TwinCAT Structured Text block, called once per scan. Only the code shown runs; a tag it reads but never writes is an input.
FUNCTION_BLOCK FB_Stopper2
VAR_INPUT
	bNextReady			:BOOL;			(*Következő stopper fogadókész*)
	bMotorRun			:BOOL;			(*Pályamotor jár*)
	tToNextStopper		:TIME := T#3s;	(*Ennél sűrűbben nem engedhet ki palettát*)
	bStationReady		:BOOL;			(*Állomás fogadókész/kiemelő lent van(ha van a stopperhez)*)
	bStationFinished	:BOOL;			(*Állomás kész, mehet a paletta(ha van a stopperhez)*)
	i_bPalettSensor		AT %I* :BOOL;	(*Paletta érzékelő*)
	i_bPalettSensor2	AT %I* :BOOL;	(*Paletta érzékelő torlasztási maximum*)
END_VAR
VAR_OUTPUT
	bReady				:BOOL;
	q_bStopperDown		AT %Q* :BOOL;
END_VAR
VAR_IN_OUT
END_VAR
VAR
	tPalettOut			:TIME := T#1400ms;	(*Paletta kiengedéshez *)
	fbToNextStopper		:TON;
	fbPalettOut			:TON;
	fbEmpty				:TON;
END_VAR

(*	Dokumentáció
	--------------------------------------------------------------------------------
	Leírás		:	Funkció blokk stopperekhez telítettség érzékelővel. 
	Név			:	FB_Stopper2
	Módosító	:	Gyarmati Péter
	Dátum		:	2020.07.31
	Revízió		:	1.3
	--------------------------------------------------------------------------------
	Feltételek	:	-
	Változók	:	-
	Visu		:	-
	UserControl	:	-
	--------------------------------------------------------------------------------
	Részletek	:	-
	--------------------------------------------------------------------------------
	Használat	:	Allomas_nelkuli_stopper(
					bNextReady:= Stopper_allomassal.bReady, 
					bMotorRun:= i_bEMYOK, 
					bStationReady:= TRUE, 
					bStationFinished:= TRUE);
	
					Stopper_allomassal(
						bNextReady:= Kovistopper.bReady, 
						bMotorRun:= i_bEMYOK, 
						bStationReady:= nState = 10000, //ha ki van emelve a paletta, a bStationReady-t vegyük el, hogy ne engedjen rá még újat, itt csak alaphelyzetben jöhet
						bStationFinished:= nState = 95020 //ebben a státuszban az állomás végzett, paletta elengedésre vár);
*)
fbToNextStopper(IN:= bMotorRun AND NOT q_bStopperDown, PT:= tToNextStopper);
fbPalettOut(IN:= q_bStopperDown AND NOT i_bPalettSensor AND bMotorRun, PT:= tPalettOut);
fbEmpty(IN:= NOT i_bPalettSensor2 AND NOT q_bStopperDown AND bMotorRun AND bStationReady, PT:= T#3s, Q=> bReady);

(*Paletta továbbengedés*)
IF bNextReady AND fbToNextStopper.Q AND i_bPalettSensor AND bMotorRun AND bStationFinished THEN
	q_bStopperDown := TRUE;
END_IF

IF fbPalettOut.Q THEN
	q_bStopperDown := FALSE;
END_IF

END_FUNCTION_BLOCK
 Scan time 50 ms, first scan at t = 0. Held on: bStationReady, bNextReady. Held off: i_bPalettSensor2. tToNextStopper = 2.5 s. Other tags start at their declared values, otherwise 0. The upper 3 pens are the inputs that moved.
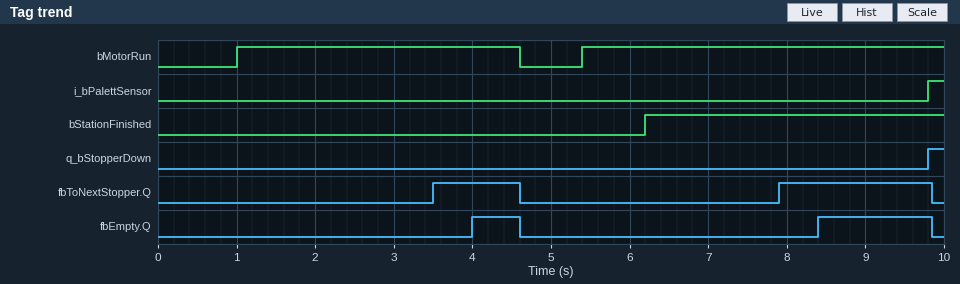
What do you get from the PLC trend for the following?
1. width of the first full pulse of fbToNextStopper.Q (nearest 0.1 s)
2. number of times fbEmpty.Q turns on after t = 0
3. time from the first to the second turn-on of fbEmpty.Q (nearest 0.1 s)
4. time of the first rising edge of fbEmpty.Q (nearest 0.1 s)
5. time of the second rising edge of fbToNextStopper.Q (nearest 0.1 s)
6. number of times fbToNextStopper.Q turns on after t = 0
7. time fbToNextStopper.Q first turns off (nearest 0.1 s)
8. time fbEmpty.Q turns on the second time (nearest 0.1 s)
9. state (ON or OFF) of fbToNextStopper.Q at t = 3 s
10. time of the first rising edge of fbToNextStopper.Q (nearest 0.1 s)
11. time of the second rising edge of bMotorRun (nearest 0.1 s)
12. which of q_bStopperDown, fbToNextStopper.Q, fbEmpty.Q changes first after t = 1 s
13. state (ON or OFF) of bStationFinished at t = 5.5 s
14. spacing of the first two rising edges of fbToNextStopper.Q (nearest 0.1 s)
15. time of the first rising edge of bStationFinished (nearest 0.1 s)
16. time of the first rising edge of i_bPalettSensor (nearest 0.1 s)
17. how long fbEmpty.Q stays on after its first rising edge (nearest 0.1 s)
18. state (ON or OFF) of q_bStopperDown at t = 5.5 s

1.1 s
2
4.4 s
4.0 s
7.9 s
2
4.6 s
8.4 s
OFF
3.5 s
5.4 s
fbToNextStopper.Q
OFF
4.4 s
6.2 s
9.8 s
0.6 s
OFF
